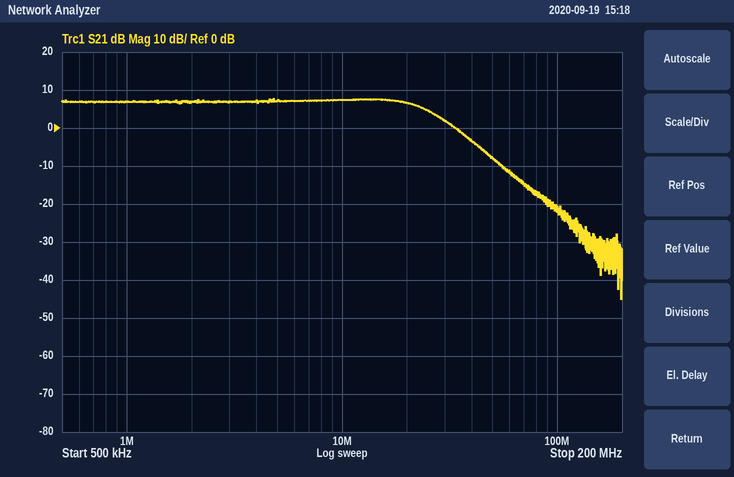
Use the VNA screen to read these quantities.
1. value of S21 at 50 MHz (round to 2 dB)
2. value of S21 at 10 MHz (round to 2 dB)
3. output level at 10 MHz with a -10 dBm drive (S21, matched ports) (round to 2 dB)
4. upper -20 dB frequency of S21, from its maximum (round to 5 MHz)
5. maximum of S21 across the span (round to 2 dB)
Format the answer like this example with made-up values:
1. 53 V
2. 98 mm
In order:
1. -8 dB
2. 8 dB
3. -2 dBm
4. 60 MHz
5. 8 dB
